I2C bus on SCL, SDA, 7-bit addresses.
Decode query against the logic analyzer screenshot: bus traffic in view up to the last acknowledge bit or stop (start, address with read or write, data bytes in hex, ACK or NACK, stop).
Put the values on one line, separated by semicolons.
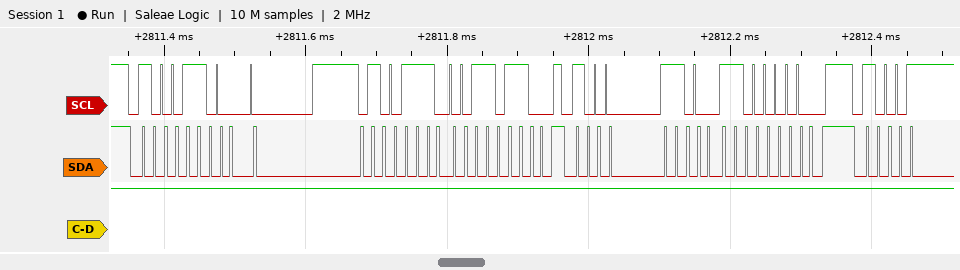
start, address 46 write ACK, 27 ACK, 36 ACK, stop, start, address 46 write ACK, C0 ACK, stop
